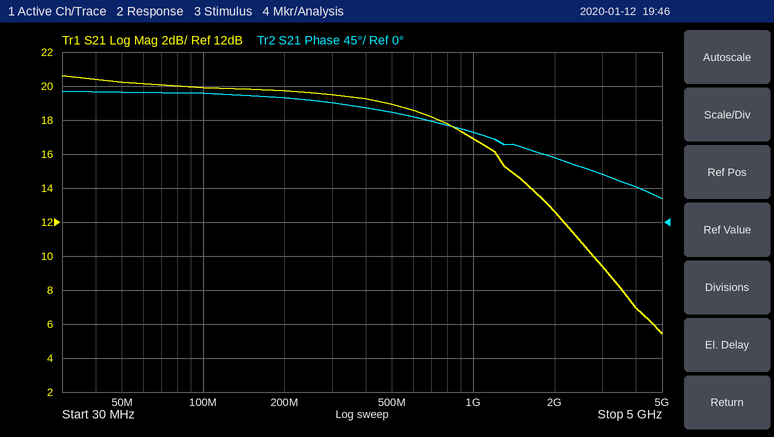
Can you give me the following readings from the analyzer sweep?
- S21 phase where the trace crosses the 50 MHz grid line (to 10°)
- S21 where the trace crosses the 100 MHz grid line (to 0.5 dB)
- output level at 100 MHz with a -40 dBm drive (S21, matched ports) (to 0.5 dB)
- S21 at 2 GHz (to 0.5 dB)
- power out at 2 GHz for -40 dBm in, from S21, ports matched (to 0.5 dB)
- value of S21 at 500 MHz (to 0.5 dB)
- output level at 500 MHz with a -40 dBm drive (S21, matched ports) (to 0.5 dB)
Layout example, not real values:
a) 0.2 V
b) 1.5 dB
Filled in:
a) 170°
b) 20.0 dB
c) -20.0 dBm
d) 12.5 dB
e) -27.5 dBm
f) 19.0 dB
g) -21.0 dBm
